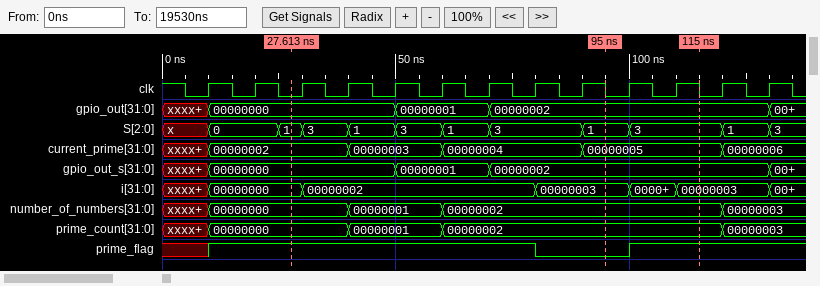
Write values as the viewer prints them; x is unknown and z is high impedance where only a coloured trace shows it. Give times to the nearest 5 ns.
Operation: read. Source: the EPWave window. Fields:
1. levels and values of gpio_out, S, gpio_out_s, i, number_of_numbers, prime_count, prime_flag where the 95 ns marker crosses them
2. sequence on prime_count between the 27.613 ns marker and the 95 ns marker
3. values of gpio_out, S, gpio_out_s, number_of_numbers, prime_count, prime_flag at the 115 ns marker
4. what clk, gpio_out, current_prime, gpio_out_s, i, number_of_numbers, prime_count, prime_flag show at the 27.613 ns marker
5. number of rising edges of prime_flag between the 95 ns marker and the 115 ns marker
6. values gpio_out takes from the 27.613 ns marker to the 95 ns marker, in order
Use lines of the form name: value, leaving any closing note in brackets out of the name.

levels and values of gpio_out, S, gpio_out_s, i, number_of_numbers, prime_count, prime_flag where the 95 ns marker crosses them: gpio_out=00000002, S=1, gpio_out_s=00000002, i=00000003, number_of_numbers=00000002, prime_count=00000002, prime_flag=0
sequence on prime_count between the 27.613 ns marker and the 95 ns marker: 00000000, 00000001, 00000002
values of gpio_out, S, gpio_out_s, number_of_numbers, prime_count, prime_flag at the 115 ns marker: gpio_out=00000002, S=3, gpio_out_s=00000002, number_of_numbers=00000002, prime_count=00000002, prime_flag=1
what clk, gpio_out, current_prime, gpio_out_s, i, number_of_numbers, prime_count, prime_flag show at the 27.613 ns marker: clk=0, gpio_out=00000000, current_prime=00000002, gpio_out_s=00000000, i=00000000, number_of_numbers=00000000, prime_count=00000000, prime_flag=1
number of rising edges of prime_flag between the 95 ns marker and the 115 ns marker: 1
values gpio_out takes from the 27.613 ns marker to the 95 ns marker, in order: 00000000, 00000001, 00000002
